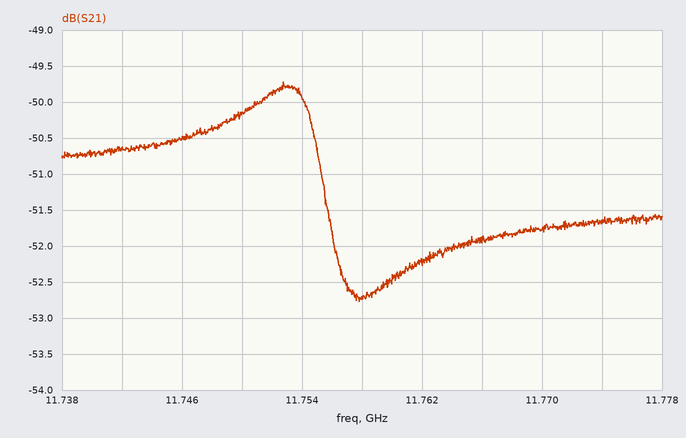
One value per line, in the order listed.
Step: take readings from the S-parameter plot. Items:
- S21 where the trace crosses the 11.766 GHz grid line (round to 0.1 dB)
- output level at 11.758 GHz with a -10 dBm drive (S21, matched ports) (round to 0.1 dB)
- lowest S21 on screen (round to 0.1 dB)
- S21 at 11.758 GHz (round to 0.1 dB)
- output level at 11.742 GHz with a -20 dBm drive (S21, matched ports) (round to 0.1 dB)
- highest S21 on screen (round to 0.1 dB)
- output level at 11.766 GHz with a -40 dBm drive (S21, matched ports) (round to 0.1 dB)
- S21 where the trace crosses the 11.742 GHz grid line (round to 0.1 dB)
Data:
-51.9 dB
-62.7 dBm
-52.8 dB
-52.7 dB
-70.6 dBm
-49.7 dB
-91.9 dBm
-50.6 dB
